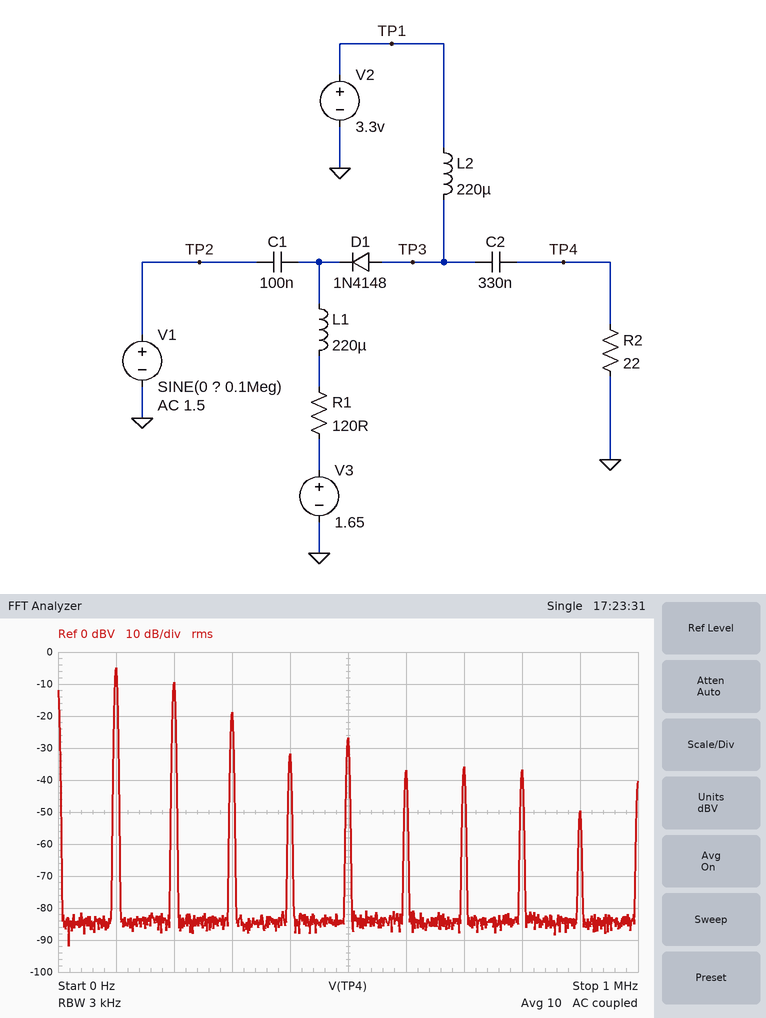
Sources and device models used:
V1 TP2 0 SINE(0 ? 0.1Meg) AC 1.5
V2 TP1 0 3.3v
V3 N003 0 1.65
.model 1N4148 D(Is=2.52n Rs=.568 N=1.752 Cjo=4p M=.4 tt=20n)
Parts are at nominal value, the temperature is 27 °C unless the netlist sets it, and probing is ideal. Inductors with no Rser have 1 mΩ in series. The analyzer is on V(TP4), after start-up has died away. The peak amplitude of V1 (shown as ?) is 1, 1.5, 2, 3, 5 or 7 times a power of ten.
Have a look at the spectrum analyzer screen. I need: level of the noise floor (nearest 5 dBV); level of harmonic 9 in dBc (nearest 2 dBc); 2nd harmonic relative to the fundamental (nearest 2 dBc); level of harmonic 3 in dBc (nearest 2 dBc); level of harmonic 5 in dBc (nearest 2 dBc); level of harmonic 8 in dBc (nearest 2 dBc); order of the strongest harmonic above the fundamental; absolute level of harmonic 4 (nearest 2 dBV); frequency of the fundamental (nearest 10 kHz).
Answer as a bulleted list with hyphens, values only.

- -85 dBV
- -44 dBc
- -4 dBc
- -14 dBc
- -22 dBc
- -32 dBc
- 2
- -32 dBV
- 100 kHz
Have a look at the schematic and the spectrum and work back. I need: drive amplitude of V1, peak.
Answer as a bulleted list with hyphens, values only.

- 3 V
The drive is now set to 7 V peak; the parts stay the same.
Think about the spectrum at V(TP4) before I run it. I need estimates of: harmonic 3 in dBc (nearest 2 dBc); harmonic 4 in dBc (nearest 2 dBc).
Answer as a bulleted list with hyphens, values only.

- -12 dBc
- -30 dBc
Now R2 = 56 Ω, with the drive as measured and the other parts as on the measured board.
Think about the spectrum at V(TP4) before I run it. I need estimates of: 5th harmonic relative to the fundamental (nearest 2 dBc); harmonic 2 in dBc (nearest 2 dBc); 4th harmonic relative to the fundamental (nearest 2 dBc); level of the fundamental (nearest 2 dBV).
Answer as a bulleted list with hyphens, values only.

- -40 dBc
- -6 dBc
- -22 dBc
- 0 dBV
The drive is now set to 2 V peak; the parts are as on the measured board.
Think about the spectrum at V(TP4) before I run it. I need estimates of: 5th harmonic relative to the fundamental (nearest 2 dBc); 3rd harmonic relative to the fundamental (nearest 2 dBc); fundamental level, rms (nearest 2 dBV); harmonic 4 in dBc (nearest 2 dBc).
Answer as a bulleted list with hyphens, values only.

- -24 dBc
- -16 dBc
- -8 dBV
- -24 dBc
